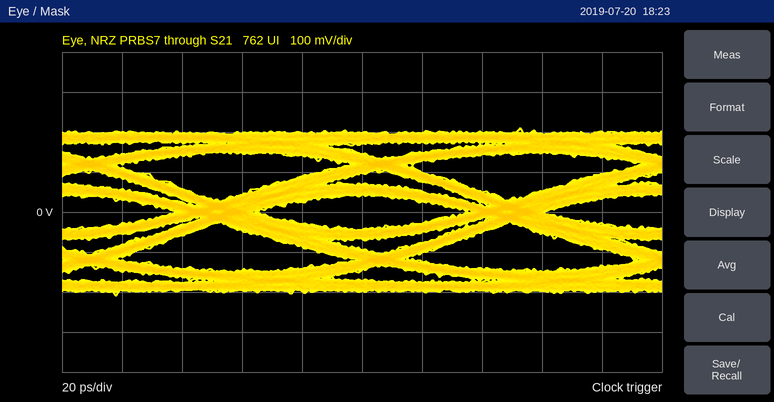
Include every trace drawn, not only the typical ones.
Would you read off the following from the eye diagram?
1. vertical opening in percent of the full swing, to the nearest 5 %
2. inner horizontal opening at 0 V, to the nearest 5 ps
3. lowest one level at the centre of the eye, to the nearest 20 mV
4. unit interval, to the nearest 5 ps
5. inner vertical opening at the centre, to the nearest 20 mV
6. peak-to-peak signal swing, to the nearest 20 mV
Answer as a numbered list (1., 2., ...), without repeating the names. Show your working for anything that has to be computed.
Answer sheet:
1. 80 mV / 420 mV ≈ 19.0 %, so 20 % to the nearest 5 %
2. 70 ps
3. 40 mV
4. 95 ps
5. 80 mV
6. 420 mV
